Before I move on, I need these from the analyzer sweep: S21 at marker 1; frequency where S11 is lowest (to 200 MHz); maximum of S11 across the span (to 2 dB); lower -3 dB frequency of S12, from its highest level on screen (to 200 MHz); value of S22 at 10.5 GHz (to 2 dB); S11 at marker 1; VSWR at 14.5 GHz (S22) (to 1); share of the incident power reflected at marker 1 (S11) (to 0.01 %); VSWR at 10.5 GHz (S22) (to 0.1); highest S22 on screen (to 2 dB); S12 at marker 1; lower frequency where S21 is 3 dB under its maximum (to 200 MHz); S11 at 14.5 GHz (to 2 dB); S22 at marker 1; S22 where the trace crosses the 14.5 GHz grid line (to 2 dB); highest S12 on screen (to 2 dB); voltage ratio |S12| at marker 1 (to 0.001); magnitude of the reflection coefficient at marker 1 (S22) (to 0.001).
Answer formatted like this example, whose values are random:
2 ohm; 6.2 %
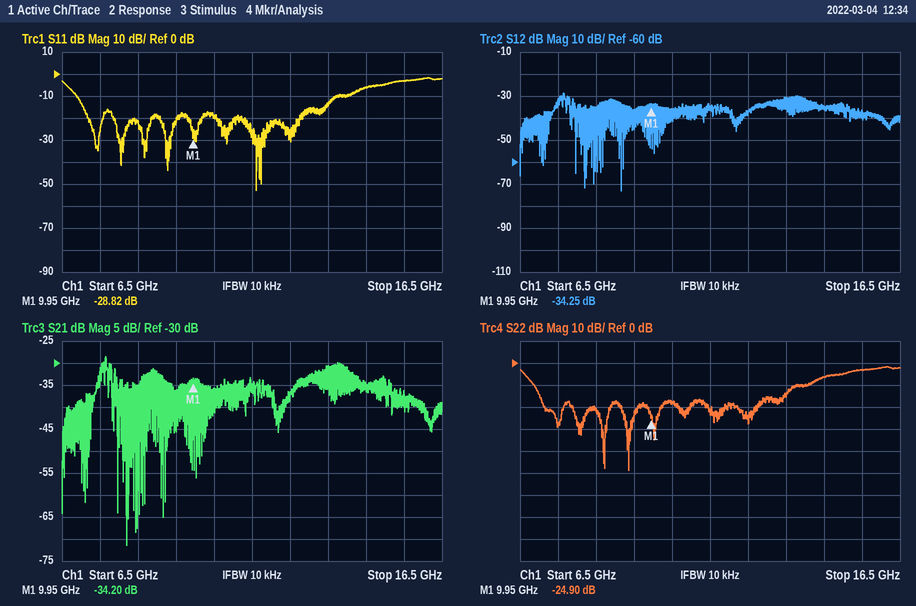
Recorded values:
-34.20 dB; 11.6 GHz; -2 dB; 7.6 GHz; -18 dB; -28.82 dB; 3; 0.13 %; 1.3; -2 dB; -34.25 dB; 7.6 GHz; -6 dB; -24.90 dB; -6 dB; -28 dB; 0.019; 0.057
